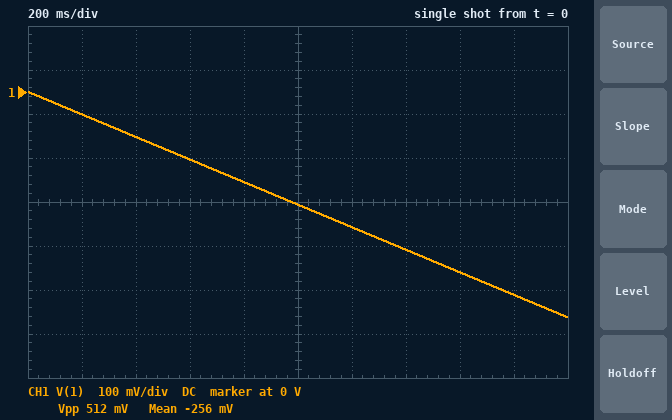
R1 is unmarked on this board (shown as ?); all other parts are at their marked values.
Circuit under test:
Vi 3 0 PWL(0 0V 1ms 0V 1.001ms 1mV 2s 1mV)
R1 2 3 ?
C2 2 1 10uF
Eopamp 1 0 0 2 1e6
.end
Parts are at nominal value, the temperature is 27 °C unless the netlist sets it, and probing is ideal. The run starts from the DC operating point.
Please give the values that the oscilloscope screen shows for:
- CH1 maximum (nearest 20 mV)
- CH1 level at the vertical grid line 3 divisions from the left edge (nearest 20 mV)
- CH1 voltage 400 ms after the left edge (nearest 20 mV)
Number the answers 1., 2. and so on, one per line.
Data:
1. 0 V
2. -160 mV
3. -100 mV
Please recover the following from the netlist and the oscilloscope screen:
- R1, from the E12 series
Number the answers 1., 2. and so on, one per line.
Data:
1. 390 Ω
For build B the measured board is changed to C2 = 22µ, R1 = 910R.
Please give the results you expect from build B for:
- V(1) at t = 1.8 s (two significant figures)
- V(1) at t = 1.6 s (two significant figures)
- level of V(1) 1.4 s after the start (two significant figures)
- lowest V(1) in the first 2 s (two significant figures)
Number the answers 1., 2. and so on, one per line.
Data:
1. -90 mV
2. -80 mV
3. -70 mV
4. -100 mV
